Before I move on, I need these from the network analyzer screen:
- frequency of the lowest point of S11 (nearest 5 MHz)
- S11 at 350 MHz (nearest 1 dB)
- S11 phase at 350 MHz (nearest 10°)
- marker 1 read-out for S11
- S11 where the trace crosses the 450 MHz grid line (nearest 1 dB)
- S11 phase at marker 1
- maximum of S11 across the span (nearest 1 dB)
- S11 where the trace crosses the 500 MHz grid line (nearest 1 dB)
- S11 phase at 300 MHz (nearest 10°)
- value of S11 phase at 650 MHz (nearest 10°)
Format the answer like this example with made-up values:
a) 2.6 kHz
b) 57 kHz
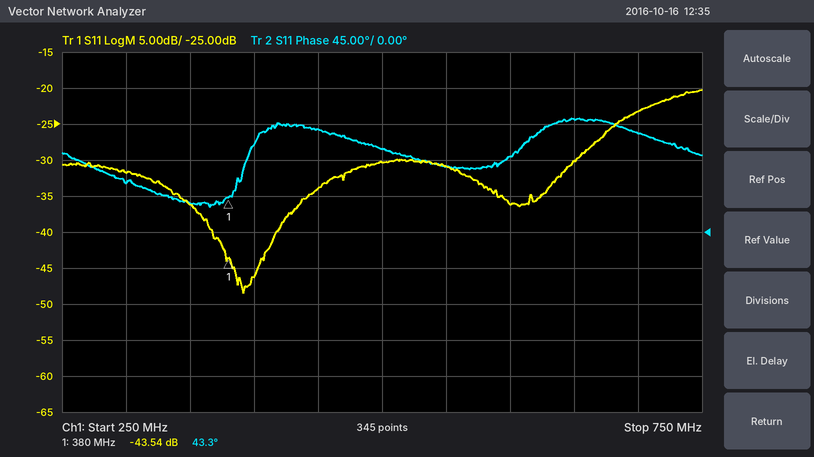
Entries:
a) 390 MHz
b) -36 dB
c) 40°
d) -43.54 dB
e) -34 dB
f) 43.3°
g) -20 dB
h) -30 dB
i) 60°
j) 140°
